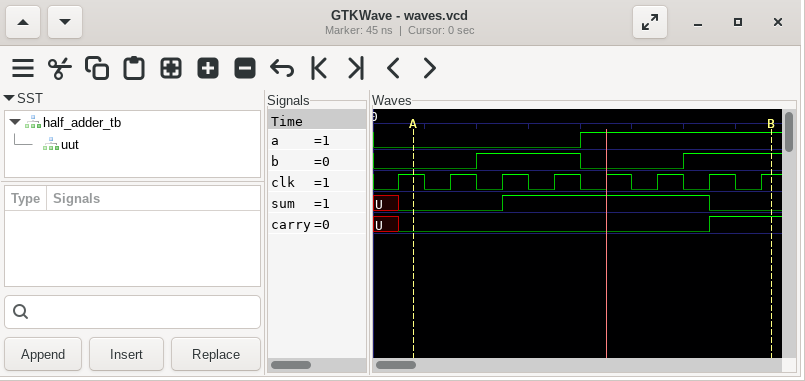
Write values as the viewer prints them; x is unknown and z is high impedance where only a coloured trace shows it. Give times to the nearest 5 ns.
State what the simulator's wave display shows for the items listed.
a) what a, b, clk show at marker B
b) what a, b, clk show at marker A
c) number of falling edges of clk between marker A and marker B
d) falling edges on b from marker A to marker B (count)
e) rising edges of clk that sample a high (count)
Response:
a=1, b=1, clk=1
a=0, b=0, clk=1
7
1
4
